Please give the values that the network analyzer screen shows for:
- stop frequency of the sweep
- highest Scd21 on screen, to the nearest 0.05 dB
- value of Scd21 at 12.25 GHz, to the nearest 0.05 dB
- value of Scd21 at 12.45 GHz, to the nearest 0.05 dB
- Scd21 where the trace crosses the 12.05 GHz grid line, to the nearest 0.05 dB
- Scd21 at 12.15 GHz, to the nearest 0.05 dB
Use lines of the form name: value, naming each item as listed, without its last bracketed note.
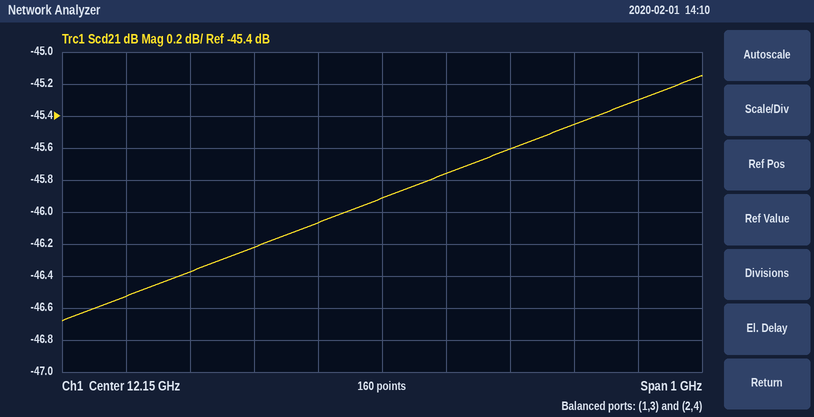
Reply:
stop frequency of the sweep: 12.65 GHz
highest Scd21 on screen, to the nearest 0.05 dB: -45.15 dB
value of Scd21 at 12.25 GHz, to the nearest 0.05 dB: -45.75 dB
value of Scd21 at 12.45 GHz, to the nearest 0.05 dB: -45.45 dB
Scd21 where the trace crosses the 12.05 GHz grid line, to the nearest 0.05 dB: -46.05 dB
Scd21 at 12.15 GHz, to the nearest 0.05 dB: -45.90 dB
